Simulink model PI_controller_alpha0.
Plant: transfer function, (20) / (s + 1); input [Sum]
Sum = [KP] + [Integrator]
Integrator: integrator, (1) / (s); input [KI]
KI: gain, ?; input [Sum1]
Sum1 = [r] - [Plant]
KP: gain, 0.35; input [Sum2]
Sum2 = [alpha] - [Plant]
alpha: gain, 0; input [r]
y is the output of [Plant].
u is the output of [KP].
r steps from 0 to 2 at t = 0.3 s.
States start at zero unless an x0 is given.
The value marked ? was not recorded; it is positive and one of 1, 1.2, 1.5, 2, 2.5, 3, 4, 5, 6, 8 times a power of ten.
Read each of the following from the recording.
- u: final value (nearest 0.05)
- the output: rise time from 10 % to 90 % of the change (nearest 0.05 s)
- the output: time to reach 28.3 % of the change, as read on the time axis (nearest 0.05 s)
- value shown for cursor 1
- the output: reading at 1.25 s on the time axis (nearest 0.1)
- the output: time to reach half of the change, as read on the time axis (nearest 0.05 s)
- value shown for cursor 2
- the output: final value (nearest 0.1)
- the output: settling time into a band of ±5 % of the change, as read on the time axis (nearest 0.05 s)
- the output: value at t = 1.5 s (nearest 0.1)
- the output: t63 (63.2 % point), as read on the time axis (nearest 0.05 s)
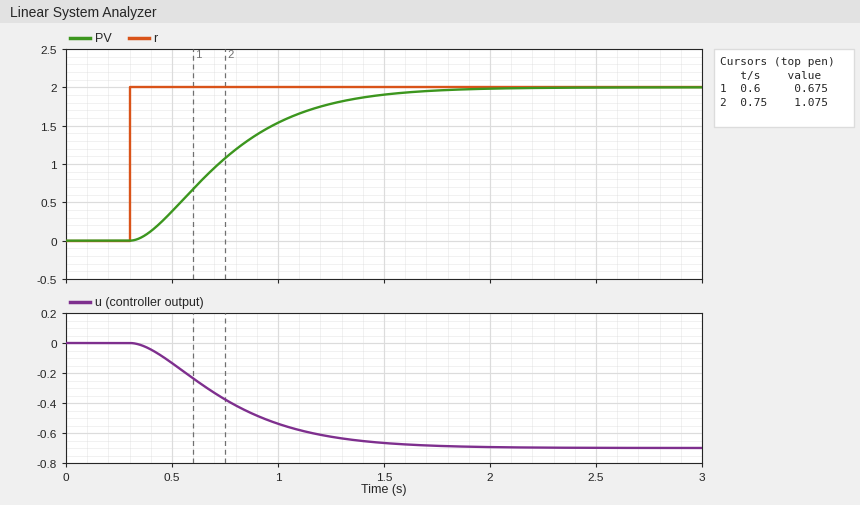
-0.70
0.85 s
0.55 s
0.675
1.8
0.70 s
1.075
2.0
1.50 s
1.9
0.85 s
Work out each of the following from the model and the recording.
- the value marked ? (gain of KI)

0.8
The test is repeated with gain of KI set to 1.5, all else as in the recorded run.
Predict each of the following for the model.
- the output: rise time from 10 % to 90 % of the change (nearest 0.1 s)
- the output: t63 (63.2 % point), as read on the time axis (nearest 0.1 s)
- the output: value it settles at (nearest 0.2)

0.4 s
0.6 s
2.0
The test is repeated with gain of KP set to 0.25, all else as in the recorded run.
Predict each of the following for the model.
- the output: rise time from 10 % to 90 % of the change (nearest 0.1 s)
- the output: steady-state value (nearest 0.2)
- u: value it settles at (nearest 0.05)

0.6 s
2.0
-0.50
